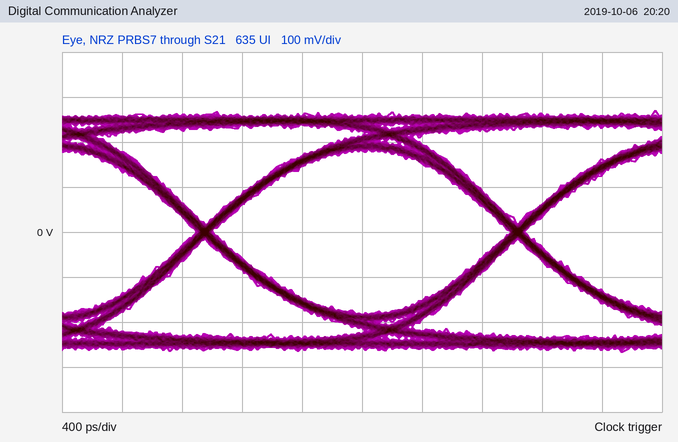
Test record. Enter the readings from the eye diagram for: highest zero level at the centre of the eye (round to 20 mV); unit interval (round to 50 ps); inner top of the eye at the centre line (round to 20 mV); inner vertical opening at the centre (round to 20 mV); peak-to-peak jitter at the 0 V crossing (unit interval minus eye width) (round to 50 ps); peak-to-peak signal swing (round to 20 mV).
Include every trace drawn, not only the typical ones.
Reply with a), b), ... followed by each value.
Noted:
a) -180 mV
b) 2.10 ns
c) 180 mV
d) 360 mV
e) 100 ps
f) 540 mV
